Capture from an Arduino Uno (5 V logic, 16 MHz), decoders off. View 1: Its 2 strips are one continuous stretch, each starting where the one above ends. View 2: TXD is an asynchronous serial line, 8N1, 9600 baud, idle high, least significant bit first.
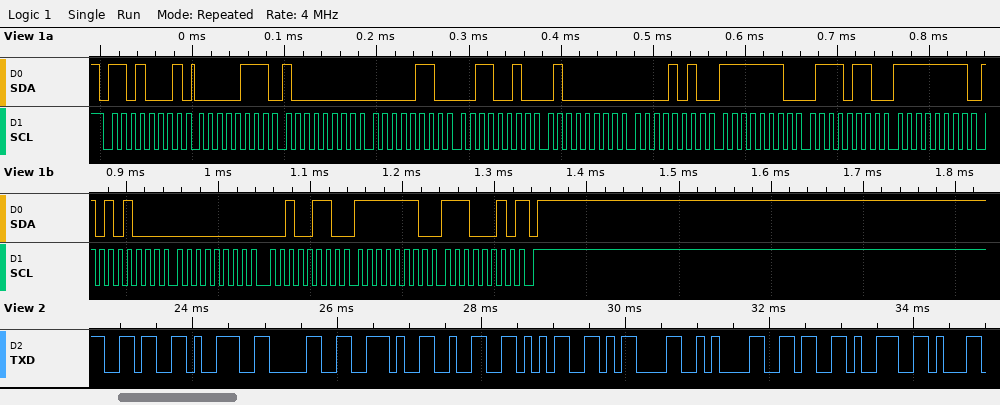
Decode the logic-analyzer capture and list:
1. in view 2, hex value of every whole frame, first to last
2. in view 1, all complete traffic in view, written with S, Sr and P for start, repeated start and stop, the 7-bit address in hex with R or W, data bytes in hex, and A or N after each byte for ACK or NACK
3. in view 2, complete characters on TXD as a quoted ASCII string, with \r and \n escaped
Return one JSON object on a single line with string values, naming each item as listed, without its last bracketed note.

{"in view 2, hex value of every whole frame, first to last": "36 39 30 2E 32 35 0D 0A 36 39", "in view 1, all complete traffic in view, written with S, Sr and P for start, repeated start and stop, the 7-bit address in hex with R or W, data bytes in hex, and A or N after each byte for ACK or NACK": "S 68R A 07 A 80 A 06 A 32 A 40 A 0A A FE A 76 A FF A A8 A 00 A 26 A FE A E2 N P", "in view 2, complete characters on TXD as a quoted ASCII string, with \\r and \\n escaped": "\"690.25\\r\\n69\""}
